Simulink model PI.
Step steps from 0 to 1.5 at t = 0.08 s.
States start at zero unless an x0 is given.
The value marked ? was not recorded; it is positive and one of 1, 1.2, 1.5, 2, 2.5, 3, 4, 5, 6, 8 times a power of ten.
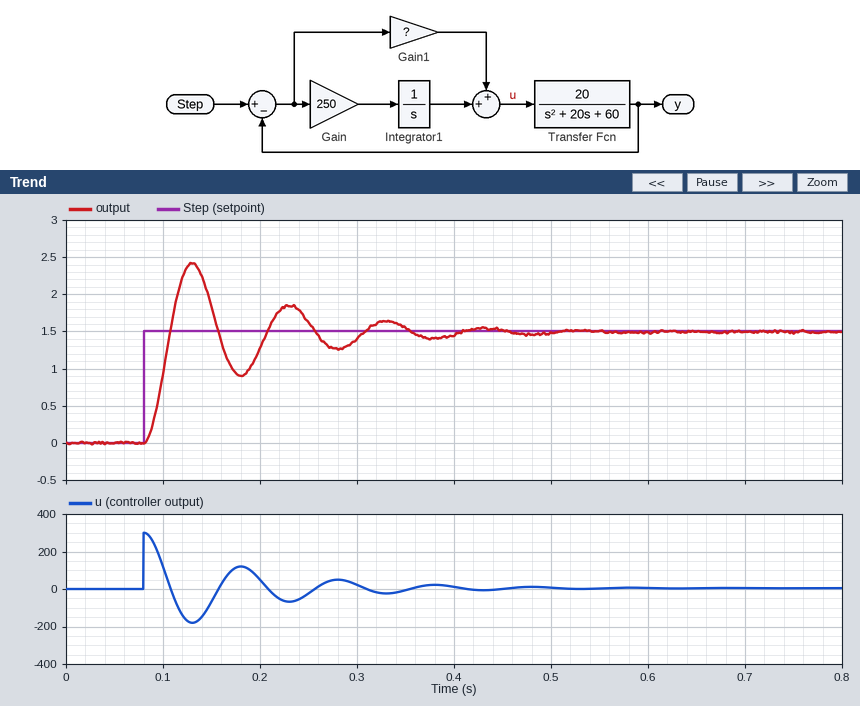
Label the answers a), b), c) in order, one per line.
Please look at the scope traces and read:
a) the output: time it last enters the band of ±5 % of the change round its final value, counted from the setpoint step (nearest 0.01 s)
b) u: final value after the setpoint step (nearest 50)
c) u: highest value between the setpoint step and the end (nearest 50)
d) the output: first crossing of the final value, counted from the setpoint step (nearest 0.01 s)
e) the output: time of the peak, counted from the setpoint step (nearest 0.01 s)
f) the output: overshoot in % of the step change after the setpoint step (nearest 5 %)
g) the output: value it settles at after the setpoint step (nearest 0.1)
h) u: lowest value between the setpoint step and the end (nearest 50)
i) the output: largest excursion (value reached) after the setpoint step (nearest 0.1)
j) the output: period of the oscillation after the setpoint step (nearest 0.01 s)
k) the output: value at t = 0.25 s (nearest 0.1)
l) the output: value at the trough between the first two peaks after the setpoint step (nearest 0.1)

a) 0.31 s
b) 0
c) 300
d) 0.03 s
e) 0.05 s
f) 60 %
g) 1.5
h) -200
i) 2.4
j) 0.10 s
k) 1.6
l) 0.9
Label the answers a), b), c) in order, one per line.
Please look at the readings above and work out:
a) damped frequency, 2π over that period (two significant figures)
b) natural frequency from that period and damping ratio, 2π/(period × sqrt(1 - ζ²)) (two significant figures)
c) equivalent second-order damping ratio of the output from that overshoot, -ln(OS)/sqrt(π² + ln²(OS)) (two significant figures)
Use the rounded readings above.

a) 63 rad/s
b) 64 rad/s
c) 0.16
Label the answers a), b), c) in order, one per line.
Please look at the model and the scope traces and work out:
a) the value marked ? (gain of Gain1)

a) 200
